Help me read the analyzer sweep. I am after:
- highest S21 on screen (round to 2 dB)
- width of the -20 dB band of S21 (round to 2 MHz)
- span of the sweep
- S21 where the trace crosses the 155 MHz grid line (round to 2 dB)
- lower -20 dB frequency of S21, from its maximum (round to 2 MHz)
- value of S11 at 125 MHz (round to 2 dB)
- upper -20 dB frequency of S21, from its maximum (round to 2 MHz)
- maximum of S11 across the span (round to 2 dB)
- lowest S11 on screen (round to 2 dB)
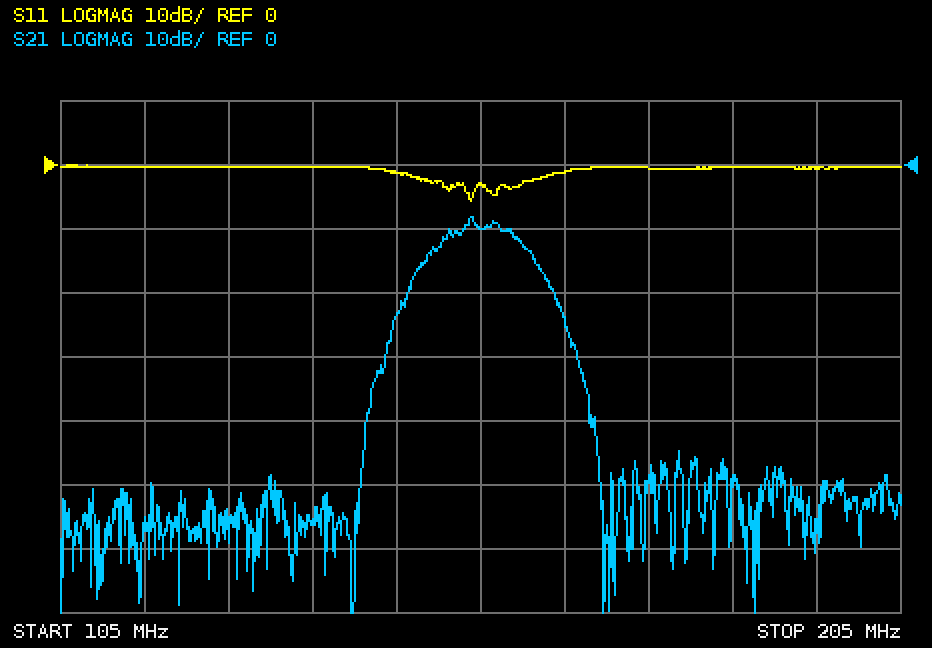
-8 dB
22 MHz
100 MHz
-10 dB
144 MHz
0 dB
166 MHz
0 dB
-6 dB
